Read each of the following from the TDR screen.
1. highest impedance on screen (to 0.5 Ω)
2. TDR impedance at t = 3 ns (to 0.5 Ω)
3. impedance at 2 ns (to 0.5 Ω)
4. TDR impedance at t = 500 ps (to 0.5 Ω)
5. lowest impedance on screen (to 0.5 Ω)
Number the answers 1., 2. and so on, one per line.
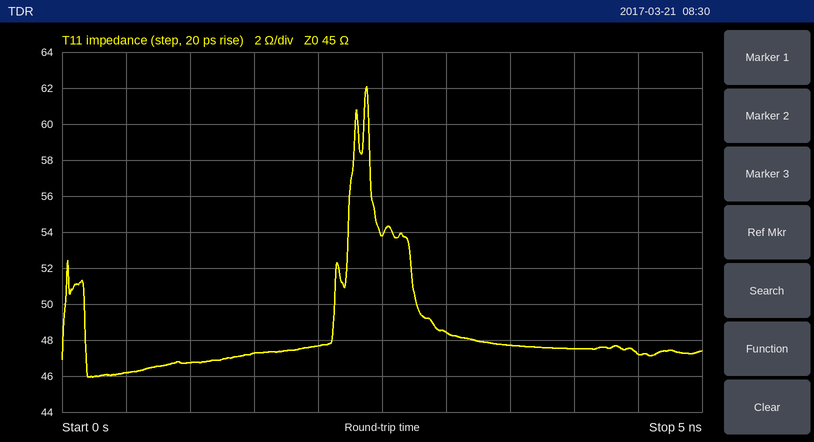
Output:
1. 62.0 Ω
2. 48.5 Ω
3. 47.5 Ω
4. 46.0 Ω
5. 46.0 Ω
